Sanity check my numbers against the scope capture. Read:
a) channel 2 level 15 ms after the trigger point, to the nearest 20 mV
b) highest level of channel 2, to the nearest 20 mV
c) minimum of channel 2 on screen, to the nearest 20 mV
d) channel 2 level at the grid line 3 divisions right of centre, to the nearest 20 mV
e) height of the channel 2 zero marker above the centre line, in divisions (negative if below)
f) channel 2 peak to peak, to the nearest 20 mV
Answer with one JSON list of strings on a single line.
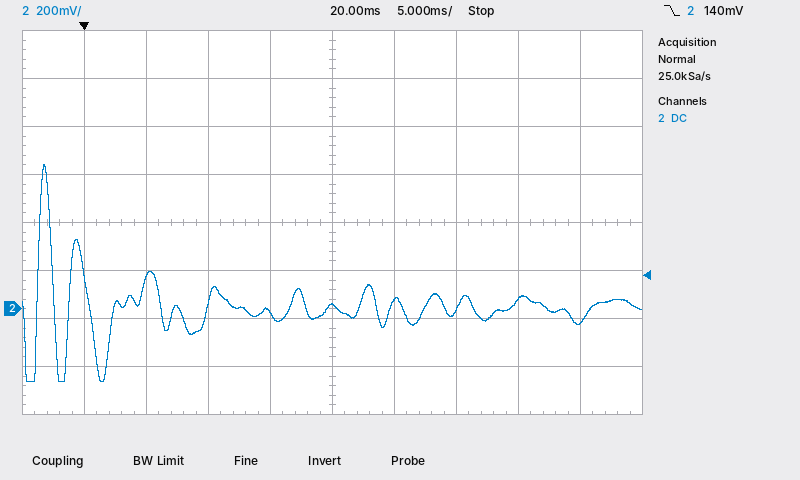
["-20 mV", "600 mV", "-300 mV", "40 mV", "-1.8 div", "900 mV"]
